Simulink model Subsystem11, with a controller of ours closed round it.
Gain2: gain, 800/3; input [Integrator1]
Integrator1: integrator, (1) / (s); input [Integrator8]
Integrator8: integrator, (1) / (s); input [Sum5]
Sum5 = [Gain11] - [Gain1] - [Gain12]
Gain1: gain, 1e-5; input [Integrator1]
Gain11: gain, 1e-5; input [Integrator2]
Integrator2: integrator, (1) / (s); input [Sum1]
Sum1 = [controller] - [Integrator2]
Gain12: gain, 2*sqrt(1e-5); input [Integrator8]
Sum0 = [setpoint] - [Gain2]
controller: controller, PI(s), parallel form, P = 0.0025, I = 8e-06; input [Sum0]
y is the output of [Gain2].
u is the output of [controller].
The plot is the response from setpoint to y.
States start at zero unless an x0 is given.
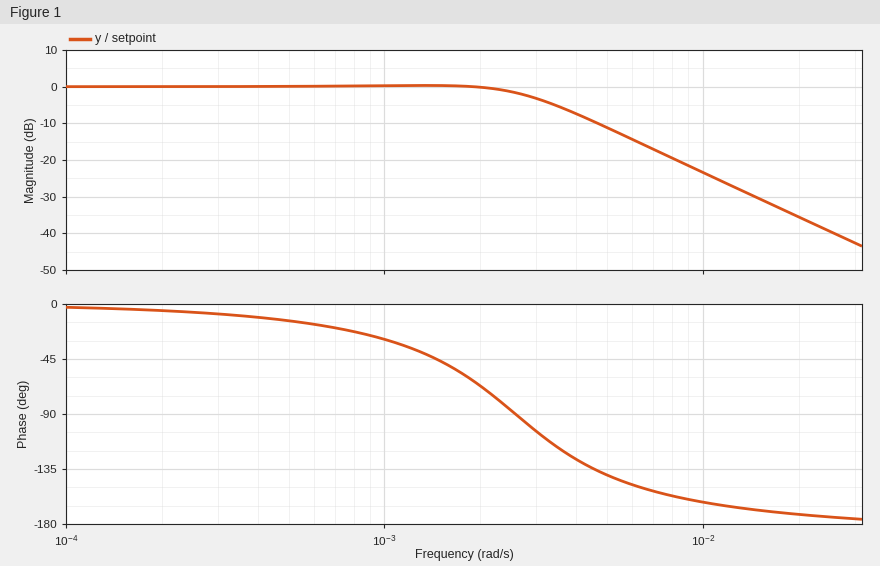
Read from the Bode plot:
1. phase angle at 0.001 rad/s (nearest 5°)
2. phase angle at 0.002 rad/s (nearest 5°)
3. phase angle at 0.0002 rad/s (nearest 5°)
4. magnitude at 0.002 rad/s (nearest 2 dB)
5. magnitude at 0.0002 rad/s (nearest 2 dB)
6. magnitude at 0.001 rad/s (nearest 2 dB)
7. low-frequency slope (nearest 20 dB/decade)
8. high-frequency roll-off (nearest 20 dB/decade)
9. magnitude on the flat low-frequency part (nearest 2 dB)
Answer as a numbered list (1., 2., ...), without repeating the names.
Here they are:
1. -30°
2. -65°
3. -5°
4. 0 dB
5. 0 dB
6. 0 dB
7. 0 dB/decade
8. -40 dB/decade
9. 0 dB
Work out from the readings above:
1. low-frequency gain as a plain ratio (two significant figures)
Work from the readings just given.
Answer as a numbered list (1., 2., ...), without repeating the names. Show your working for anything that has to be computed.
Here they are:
1. 10^(0 / 20) = 1.0
